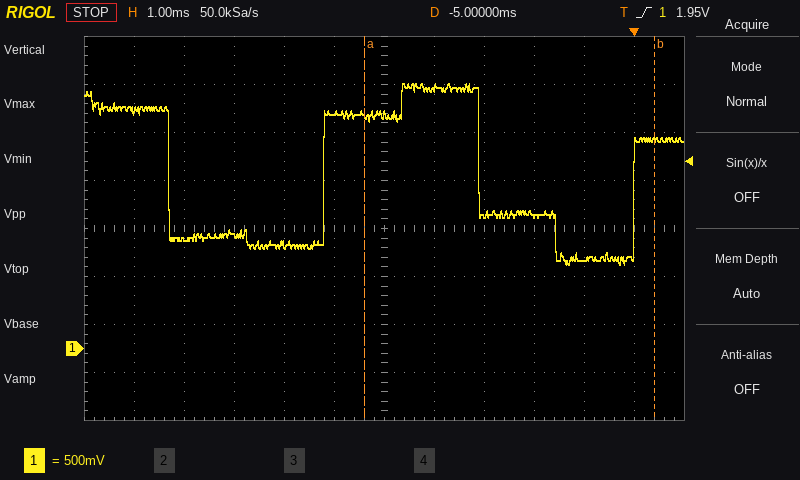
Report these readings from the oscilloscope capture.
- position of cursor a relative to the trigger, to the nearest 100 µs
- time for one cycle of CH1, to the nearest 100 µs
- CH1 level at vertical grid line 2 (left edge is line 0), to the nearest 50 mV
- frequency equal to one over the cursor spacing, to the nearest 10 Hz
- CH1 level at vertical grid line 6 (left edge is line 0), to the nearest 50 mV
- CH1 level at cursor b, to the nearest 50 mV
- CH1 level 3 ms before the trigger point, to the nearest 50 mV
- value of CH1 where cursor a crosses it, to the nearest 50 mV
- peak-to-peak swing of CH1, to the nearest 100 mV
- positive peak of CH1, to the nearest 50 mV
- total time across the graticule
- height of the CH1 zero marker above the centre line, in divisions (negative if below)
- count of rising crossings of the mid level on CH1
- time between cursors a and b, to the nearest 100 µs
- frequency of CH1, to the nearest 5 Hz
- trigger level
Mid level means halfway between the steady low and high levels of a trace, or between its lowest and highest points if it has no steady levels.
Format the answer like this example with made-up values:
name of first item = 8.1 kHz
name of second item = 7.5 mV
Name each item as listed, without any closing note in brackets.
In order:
position of cursor a relative to the trigger, to the nearest 100 µs = -5.4 ms
time for one cycle of CH1, to the nearest 100 µs = 6.2 ms
CH1 level at vertical grid line 2 (left edge is line 0), to the nearest 50 mV = 1.15 V
frequency equal to one over the cursor spacing, to the nearest 10 Hz = 170 Hz
CH1 level at vertical grid line 6 (left edge is line 0), to the nearest 50 mV = 2.45 V
CH1 level at cursor b, to the nearest 50 mV = 2.20 V
CH1 level 3 ms before the trigger point, to the nearest 50 mV = 1.40 V
value of CH1 where cursor a crosses it, to the nearest 50 mV = 2.45 V
peak-to-peak swing of CH1, to the nearest 100 mV = 1.90 V
positive peak of CH1, to the nearest 50 mV = 2.75 V
total time across the graticule = 12 ms
height of the CH1 zero marker above the centre line, in divisions = -2.5 div
count of rising crossings of the mid level on CH1 = 2
time between cursors a and b, to the nearest 100 µs = 5.8 ms
frequency of CH1, to the nearest 5 Hz = 160 Hz
trigger level = 1.95 V
